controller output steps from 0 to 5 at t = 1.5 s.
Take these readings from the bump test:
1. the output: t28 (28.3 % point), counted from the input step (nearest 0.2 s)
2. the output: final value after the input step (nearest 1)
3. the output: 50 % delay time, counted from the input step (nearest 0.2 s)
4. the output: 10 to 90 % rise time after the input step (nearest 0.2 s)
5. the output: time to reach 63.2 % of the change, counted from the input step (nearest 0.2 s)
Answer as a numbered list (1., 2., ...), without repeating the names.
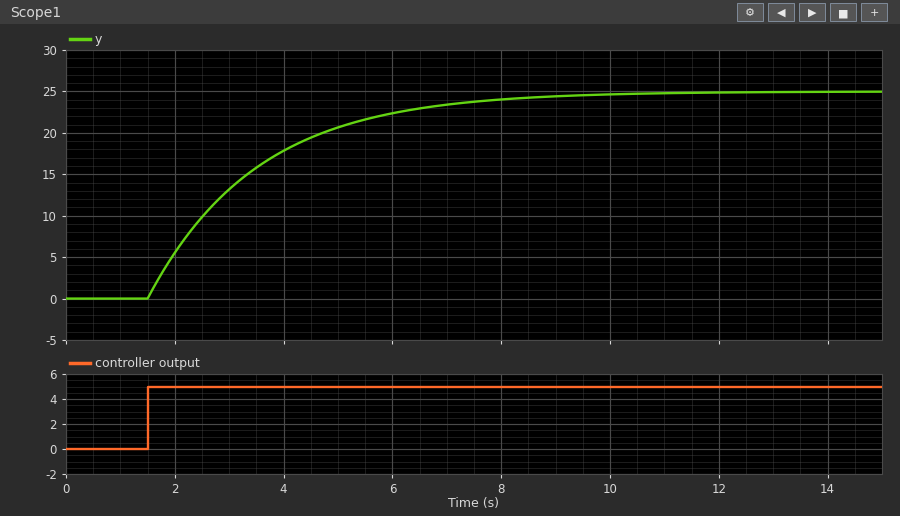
1. 0.6 s
2. 25
3. 1.4 s
4. 4.4 s
5. 2.0 s
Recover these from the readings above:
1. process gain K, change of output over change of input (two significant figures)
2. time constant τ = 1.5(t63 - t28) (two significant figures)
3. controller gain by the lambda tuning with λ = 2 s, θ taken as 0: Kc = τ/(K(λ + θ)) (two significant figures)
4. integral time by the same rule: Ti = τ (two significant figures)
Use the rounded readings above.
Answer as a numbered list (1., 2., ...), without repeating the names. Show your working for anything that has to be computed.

1. (25 - 0) / 5 = 5.0
2. 1.5 × (2 - 0.6) = 2.1 s
3. 2.1 / (5 × (2 + 0)) = 0.21
4. 2.1 s
